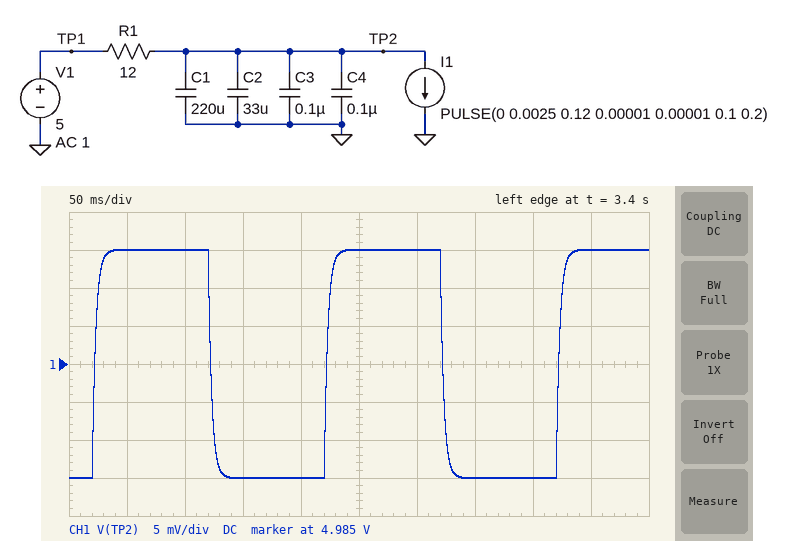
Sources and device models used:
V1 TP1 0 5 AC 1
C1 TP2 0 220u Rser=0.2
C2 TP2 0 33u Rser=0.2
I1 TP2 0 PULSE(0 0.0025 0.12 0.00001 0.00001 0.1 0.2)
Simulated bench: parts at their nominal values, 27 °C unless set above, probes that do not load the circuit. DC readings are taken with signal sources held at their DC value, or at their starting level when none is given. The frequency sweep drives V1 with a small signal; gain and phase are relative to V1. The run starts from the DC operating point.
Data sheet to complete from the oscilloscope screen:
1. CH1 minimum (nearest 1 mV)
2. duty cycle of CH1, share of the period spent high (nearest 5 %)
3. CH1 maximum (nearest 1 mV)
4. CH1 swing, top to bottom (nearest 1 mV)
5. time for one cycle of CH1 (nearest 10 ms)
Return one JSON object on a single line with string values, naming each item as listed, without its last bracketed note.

{"CH1 minimum": "4.970 V", "duty cycle of CH1, share of the period spent high": "50 %", "CH1 maximum": "5.000 V", "CH1 swing, top to bottom": "30 mV", "time for one cycle of CH1": "200 ms"}
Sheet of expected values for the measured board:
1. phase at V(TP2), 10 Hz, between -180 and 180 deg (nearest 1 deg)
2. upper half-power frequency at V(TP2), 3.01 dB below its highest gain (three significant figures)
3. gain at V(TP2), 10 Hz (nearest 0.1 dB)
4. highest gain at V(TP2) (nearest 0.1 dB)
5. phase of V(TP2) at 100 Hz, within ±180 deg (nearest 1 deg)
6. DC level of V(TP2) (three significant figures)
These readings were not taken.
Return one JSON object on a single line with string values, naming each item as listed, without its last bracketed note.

{"phase at V(TP2), 10 Hz, between -180 and 180 deg": "-11 deg", "upper half-power frequency at V(TP2), 3.01 dB below its highest gain": "51.7 Hz", "gain at V(TP2), 10 Hz": "-0.2 dB", "highest gain at V(TP2)": "0 dB", "phase of V(TP2) at 100 Hz, within ±180 deg": "-61 deg", "DC level of V(TP2)": "5.00 V"}
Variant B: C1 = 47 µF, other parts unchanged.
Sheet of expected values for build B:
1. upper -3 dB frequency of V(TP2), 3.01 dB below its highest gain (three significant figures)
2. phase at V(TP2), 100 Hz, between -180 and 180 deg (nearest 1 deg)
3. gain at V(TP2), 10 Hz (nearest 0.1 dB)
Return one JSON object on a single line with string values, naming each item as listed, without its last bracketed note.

{"upper -3 dB frequency of V(TP2), 3.01 dB below its highest gain": "164 Hz", "phase at V(TP2), 100 Hz, between -180 and 180 deg": "-31 deg", "gain at V(TP2), 10 Hz": "0 dB"}
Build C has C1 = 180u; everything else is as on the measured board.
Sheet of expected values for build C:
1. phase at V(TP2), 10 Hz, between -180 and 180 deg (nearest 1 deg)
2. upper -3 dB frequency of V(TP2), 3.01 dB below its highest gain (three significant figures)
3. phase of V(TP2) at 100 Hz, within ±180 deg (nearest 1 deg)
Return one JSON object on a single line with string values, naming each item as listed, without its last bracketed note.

{"phase at V(TP2), 10 Hz, between -180 and 180 deg": "-9 deg", "upper -3 dB frequency of V(TP2), 3.01 dB below its highest gain": "61.5 Hz", "phase of V(TP2) at 100 Hz, within ±180 deg": "-57 deg"}
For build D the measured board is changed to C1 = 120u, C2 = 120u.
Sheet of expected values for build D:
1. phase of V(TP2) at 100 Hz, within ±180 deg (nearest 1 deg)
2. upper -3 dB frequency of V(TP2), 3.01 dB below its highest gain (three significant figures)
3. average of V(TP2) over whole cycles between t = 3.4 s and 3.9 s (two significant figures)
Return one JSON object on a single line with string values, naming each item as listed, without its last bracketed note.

{"phase of V(TP2) at 100 Hz, within ±180 deg": "-60 deg", "upper -3 dB frequency of V(TP2), 3.01 dB below its highest gain": "54.8 Hz", "average of V(TP2) over whole cycles between t = 3.4 s and 3.9 s": "5.0 V"}
